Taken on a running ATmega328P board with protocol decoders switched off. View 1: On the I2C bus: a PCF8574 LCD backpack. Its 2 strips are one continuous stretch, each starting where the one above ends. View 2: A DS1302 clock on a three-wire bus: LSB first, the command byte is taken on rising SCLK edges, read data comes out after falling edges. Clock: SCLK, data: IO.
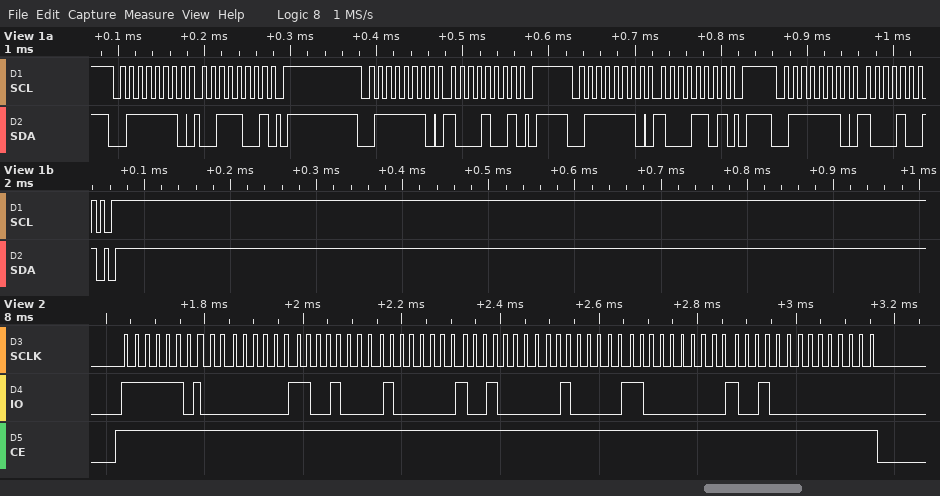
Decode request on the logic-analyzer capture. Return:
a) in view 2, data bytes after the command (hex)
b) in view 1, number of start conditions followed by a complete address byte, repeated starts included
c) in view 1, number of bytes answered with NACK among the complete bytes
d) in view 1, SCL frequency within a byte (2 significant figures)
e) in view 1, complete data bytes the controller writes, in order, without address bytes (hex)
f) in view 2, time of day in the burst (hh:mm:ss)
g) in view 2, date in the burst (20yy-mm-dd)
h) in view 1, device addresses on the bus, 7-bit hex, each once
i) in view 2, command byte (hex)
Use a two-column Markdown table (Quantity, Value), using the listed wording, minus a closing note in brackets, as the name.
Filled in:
| Quantity | Value |
|---|---|
| in view 2, data bytes after the command | 00 13 02 09 04 03 24 00 |
| in view 1, number of start conditions followed by a complete address byte, repeated starts included | 4 |
| in view 1, number of bytes answered with NACK among the complete bytes | 0 |
| in view 1, SCL frequency within a byte | 100 kHz |
| in view 1, complete data bytes the controller writes, in order, without address bytes | 39 89 8D 89 |
| in view 2, time of day in the burst | 02:13:00 |
| in view 2, date in the burst | 2024-04-09 |
| in view 1, device addresses on the bus, 7-bit hex, each once | 0x3F |
| in view 2, command byte | 0xBF |
